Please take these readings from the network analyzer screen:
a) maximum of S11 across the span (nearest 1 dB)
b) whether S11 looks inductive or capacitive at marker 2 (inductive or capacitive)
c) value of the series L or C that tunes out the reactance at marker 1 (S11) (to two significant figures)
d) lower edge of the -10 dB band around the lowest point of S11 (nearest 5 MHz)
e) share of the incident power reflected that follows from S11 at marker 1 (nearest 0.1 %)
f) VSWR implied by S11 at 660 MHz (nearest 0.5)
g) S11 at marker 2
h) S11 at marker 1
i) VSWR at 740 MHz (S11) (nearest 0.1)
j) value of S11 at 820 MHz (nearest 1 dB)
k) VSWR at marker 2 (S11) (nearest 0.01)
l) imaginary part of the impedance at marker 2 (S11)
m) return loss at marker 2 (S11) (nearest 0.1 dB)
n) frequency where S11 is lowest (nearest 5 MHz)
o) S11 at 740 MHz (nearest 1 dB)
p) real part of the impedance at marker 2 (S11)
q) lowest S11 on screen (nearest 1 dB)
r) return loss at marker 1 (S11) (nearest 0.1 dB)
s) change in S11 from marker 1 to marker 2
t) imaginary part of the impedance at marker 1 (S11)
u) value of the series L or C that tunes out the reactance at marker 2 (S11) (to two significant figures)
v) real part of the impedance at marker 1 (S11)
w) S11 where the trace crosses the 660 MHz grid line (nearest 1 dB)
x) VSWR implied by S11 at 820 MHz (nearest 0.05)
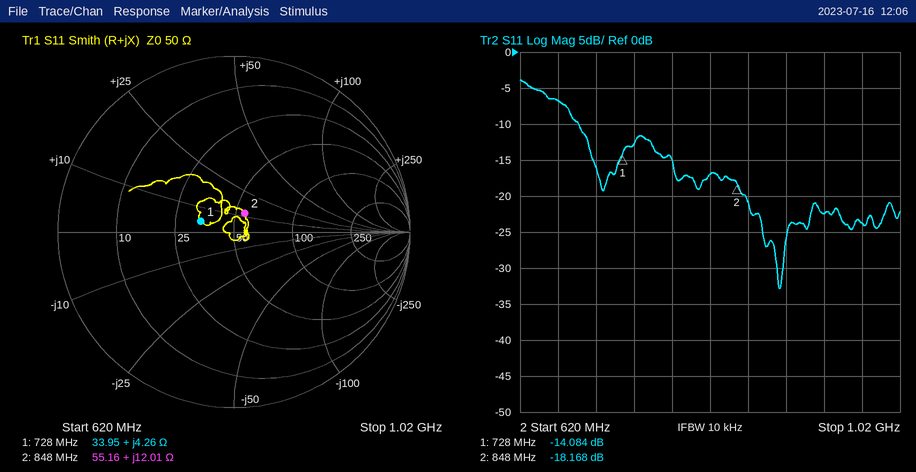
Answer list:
-4 dB
inductive
51 pF
680 MHz
3.9 %
2.5
-18.168 dB
-14.084 dB
1.6
-17 dB
1.28
+12.01 Ω
18.2 dB
895 MHz
-13 dB
55.16 Ω
-33 dB
14.1 dB
-4.084 dB
+4.26 Ω
16 pF
33.95 Ω
-7 dB
1.35
